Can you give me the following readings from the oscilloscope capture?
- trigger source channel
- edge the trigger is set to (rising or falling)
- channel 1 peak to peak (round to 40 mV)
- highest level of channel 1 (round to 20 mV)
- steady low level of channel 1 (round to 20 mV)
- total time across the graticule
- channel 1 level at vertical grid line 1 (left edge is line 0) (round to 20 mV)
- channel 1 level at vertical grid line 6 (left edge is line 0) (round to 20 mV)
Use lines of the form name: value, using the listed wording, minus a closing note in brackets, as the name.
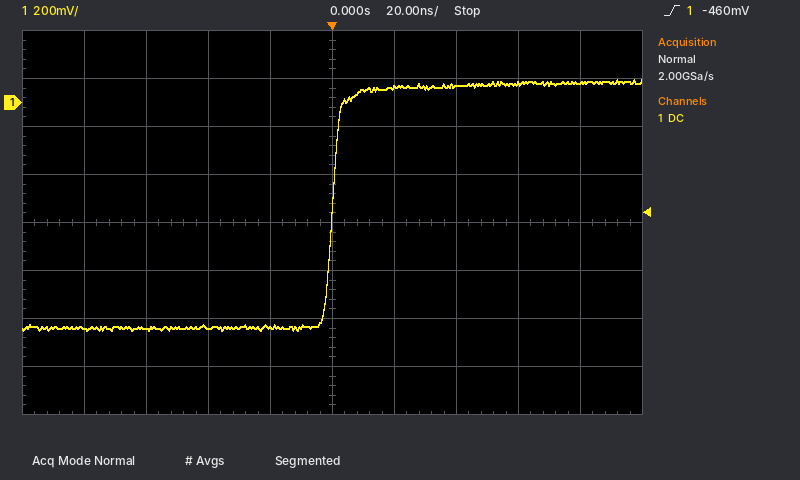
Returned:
trigger source channel: channel 1
edge the trigger is set to: rising
channel 1 peak to peak: 1.04 V
highest level of channel 1: 100 mV
steady low level of channel 1: -940 mV
total time across the graticule: 200 ns
channel 1 level at vertical grid line 1 (left edge is line 0): -940 mV
channel 1 level at vertical grid line 6 (left edge is line 0): 60 mV
